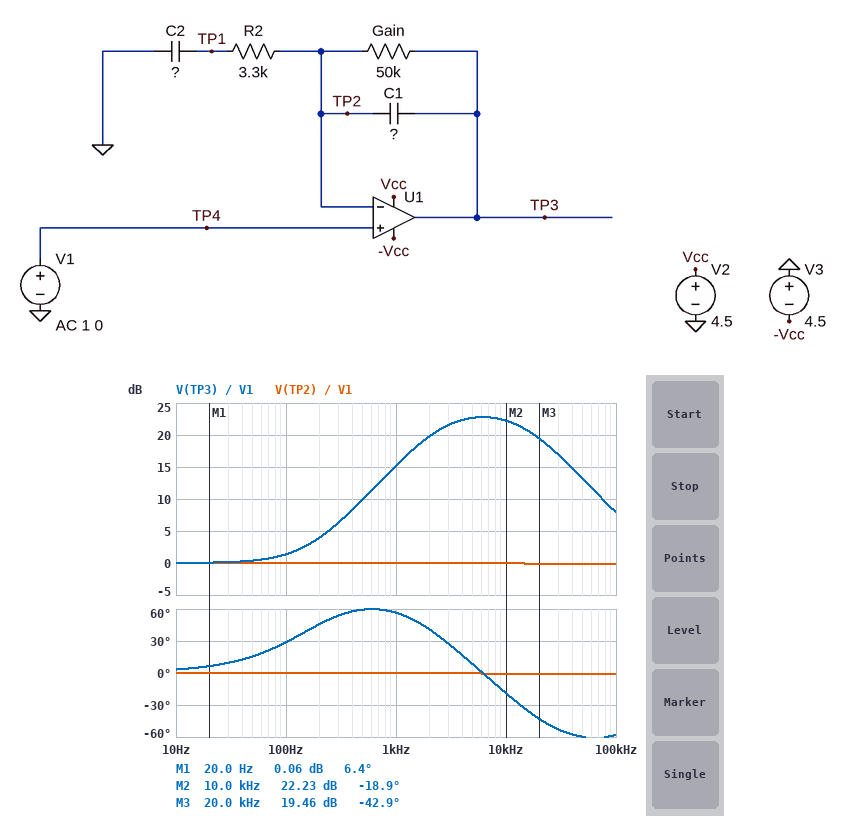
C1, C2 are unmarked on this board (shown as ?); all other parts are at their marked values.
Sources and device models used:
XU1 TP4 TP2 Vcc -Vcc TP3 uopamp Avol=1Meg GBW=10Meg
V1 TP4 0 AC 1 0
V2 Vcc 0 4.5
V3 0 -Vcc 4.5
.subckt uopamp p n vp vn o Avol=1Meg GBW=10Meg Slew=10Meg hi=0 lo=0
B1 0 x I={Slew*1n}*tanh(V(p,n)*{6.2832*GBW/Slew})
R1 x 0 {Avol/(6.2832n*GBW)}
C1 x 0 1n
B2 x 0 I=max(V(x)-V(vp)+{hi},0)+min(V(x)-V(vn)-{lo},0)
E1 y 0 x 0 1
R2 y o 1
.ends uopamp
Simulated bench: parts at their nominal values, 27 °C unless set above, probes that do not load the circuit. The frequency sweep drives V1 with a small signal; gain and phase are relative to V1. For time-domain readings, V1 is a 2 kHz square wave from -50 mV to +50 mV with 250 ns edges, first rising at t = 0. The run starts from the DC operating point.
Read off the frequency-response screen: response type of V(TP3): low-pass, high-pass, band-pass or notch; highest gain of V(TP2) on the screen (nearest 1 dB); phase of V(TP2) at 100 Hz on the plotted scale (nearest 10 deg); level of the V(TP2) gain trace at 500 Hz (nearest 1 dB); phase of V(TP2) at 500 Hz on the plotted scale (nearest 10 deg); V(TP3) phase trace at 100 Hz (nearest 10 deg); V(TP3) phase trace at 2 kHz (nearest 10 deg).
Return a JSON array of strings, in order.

["band-pass", "0 dB", "0 deg", "0 dB", "0 deg", "30 deg", "40 deg"]
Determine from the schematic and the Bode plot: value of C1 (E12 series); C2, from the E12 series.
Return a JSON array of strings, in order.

["220 pF", "18 nF"]
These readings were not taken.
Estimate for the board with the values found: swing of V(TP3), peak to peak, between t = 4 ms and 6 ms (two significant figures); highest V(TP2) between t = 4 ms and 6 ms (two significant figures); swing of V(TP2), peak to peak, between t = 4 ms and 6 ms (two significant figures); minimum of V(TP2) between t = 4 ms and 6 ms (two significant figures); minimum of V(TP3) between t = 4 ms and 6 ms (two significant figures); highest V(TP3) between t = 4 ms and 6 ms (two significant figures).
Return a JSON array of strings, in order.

["2.1 V", "50 mV", "100 mV", "-50 mV", "-1.1 V", "1.1 V"]
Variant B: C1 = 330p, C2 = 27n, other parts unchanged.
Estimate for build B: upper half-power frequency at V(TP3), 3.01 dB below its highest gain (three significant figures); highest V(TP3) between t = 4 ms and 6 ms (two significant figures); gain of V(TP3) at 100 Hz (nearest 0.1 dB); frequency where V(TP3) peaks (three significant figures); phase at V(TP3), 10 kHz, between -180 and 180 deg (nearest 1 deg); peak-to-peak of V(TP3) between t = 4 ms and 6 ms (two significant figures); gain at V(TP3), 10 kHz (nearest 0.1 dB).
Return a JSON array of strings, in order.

["12.7 kHz", "1.0 V", "2.6 dB", "4.12 kHz", "-33 deg", "2.0 V", "20.9 dB"]
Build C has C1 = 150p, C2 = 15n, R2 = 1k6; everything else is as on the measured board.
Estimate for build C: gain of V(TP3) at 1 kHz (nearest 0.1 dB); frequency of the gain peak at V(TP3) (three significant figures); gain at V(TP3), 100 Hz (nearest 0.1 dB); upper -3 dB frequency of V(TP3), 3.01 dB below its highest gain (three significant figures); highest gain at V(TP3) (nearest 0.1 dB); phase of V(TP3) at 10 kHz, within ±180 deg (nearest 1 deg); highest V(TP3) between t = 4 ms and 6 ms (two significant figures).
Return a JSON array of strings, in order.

["13.9 dB", "11.5 kHz", "0.9 dB", "30.5 kHz", "27.9 dB", "7 deg", "1.9 V"]
